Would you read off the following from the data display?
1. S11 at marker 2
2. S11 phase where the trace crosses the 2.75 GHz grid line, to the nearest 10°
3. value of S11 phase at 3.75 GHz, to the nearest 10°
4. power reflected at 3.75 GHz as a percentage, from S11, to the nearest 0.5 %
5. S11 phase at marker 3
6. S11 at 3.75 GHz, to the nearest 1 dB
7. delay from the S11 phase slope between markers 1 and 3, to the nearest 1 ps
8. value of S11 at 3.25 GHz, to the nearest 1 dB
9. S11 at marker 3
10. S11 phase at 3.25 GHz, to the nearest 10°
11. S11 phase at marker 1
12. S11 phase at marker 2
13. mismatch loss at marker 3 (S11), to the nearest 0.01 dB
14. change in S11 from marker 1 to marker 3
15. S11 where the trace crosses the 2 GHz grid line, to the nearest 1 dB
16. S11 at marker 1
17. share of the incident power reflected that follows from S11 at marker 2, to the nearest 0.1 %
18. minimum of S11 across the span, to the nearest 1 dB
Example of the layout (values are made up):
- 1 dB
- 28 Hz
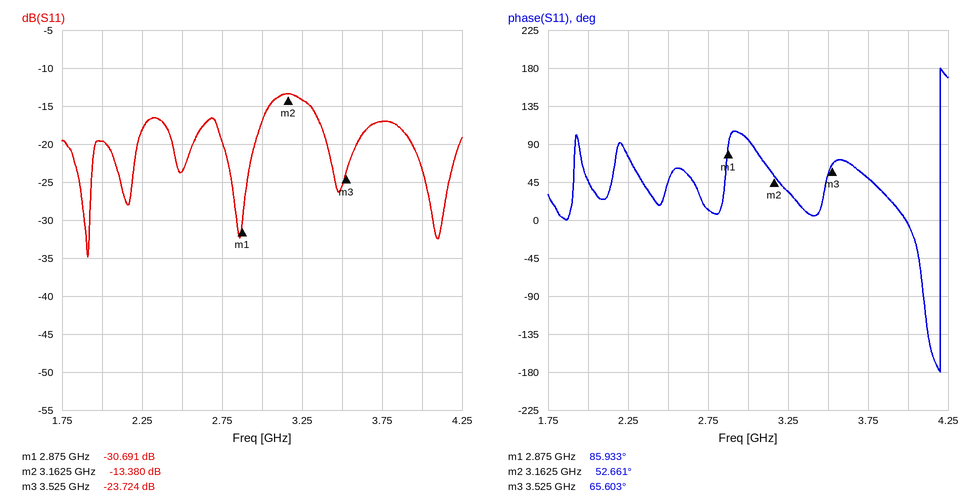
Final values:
- -13.380 dB
- 10°
- 50°
- 2.0 %
- 65.603°
- -17 dB
- 87 ps
- -14 dB
- -23.724 dB
- 30°
- 85.933°
- 52.661°
- 0.02 dB
- 6.967 dB
- -20 dB
- -30.691 dB
- 4.6 %
- -35 dB
